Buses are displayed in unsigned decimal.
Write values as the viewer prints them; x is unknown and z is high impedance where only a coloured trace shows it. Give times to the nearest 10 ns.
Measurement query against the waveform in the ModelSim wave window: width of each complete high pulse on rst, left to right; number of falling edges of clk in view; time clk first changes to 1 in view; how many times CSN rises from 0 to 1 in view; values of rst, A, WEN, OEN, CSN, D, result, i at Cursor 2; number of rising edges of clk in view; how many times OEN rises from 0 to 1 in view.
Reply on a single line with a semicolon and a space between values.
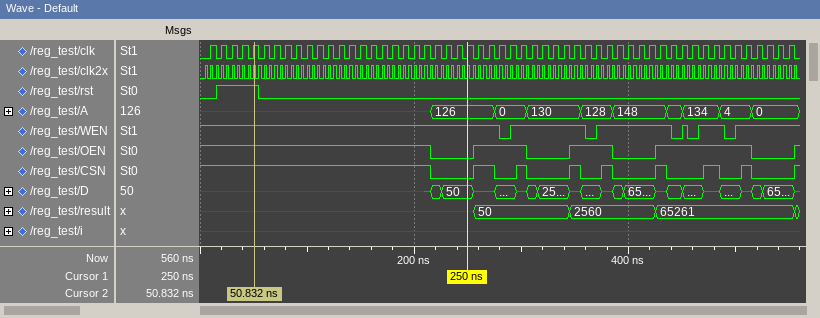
40 ns; 55; 10 ns; 8; rst=1, A=x, WEN=1, OEN=1, CSN=1, D=x, result=x, i=x; 55; 4
